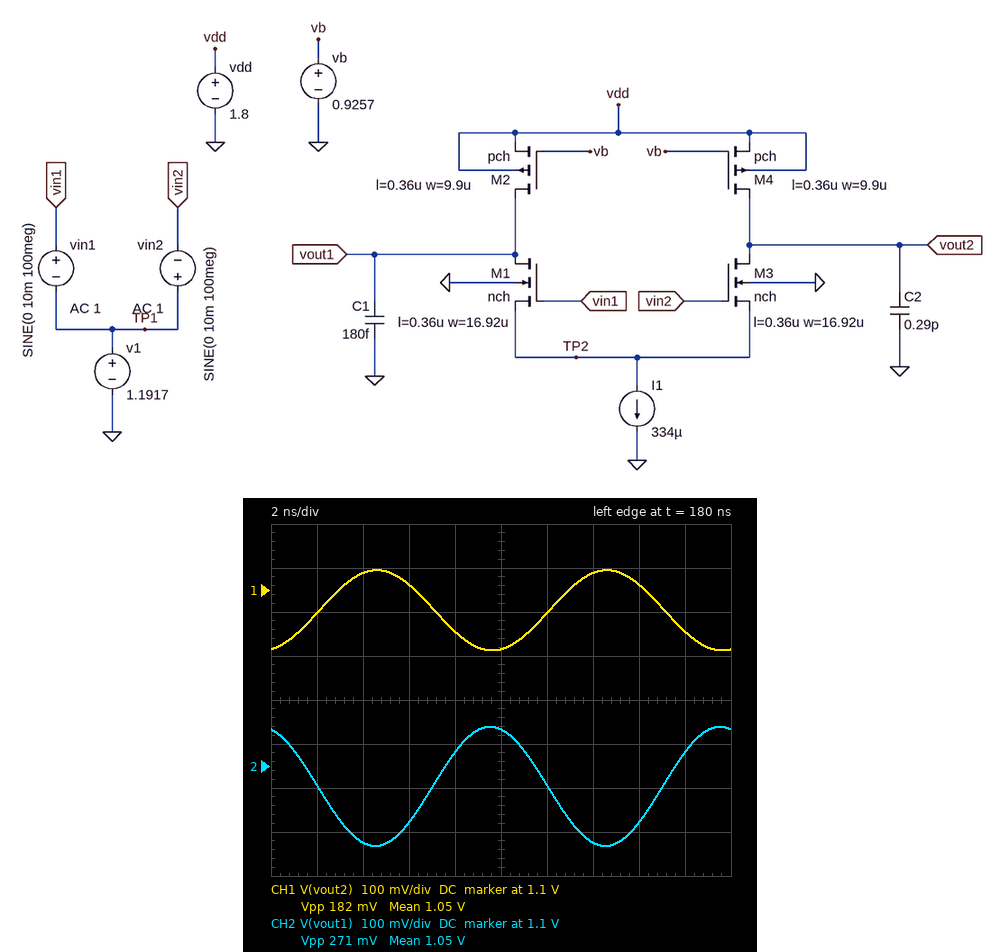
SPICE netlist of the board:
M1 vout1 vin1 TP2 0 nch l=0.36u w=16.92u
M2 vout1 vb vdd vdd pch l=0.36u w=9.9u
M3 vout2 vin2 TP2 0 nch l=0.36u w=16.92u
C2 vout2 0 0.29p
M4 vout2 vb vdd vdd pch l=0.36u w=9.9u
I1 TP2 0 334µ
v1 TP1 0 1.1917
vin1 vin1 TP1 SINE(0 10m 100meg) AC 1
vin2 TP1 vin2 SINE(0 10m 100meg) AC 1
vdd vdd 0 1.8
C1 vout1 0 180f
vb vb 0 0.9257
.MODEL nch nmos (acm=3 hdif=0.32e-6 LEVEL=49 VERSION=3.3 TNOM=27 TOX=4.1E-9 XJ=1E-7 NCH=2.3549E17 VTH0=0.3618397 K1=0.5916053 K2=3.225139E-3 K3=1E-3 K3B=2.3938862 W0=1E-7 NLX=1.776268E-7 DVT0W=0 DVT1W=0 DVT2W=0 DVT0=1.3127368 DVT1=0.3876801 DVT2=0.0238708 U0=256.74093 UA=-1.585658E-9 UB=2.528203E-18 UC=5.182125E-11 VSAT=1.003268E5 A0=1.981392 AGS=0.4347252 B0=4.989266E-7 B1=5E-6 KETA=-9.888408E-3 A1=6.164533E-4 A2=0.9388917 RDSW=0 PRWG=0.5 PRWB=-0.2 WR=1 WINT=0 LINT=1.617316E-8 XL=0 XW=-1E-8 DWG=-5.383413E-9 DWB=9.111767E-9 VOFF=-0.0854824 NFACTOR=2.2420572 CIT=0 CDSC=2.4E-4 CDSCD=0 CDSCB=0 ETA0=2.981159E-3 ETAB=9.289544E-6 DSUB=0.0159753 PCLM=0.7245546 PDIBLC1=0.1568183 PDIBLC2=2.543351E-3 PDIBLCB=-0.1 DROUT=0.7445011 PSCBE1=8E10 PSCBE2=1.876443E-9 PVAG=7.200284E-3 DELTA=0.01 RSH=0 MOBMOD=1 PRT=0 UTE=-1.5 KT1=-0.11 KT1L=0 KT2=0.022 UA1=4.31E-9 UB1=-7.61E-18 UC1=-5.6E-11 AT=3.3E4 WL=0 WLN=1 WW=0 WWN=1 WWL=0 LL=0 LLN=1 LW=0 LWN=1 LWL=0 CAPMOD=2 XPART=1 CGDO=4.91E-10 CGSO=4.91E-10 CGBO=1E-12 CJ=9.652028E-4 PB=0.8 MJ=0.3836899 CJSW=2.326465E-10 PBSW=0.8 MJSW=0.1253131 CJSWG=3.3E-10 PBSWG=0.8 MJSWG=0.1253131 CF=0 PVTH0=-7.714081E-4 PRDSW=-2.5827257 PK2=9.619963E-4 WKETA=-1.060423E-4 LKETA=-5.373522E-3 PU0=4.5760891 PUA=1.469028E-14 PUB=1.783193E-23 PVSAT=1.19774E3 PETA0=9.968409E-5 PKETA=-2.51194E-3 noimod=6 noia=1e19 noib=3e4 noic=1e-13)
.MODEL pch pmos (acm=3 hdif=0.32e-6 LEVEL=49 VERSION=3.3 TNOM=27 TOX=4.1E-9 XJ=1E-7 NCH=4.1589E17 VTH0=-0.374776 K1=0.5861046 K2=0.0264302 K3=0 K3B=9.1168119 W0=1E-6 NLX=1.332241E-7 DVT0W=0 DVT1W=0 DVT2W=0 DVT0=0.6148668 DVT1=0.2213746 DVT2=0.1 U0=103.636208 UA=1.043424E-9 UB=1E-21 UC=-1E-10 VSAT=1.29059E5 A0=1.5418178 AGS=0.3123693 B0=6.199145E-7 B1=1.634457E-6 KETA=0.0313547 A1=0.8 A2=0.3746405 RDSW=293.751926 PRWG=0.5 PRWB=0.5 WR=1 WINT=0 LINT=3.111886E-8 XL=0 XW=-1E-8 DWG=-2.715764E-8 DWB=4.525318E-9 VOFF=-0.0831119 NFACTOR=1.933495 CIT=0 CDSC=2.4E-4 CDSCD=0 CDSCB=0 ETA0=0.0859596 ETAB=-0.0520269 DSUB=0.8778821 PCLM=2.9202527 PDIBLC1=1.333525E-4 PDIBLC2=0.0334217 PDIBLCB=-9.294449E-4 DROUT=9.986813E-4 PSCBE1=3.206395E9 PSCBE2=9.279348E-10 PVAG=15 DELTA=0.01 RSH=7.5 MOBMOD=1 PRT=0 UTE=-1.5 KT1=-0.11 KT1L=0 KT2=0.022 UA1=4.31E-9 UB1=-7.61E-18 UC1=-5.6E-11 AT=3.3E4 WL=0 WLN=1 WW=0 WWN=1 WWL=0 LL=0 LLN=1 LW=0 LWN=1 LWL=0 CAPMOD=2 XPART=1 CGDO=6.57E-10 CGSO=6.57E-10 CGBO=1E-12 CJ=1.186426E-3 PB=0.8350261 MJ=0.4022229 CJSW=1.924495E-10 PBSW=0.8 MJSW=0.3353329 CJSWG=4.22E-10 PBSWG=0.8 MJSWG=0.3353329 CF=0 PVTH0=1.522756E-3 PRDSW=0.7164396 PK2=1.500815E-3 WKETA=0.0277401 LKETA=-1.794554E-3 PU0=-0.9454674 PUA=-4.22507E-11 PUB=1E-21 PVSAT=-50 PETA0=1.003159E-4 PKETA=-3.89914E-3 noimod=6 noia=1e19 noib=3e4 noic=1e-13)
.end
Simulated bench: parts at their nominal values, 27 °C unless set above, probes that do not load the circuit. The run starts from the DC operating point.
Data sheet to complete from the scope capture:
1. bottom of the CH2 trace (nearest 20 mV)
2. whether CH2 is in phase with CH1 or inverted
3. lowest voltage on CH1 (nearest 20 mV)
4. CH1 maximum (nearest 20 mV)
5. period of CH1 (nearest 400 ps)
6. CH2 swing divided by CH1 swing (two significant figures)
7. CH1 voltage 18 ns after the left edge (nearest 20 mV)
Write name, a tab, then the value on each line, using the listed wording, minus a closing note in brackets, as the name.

bottom of the CH2 trace	920 mV
whether CH2 is in phase with CH1 or inverted	inverted
lowest voltage on CH1	960 mV
CH1 maximum	1.14 V
period of CH1	10.0 ns
CH2 swing divided by CH1 swing	1.5
CH1 voltage 18 ns after the left edge	1.00 V
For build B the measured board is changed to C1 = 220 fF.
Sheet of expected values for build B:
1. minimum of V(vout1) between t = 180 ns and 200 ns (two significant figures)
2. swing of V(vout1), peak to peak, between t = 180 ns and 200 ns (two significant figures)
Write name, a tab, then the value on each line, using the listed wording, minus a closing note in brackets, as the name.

minimum of V(vout1) between t = 180 ns and 200 ns	940 mV
swing of V(vout1), peak to peak, between t = 180 ns and 200 ns	230 mV
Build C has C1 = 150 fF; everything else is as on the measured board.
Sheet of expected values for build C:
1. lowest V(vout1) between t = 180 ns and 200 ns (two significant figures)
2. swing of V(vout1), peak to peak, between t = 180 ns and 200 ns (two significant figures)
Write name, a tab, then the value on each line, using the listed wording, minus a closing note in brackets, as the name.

lowest V(vout1) between t = 180 ns and 200 ns	900 mV
swing of V(vout1), peak to peak, between t = 180 ns and 200 ns	310 mV
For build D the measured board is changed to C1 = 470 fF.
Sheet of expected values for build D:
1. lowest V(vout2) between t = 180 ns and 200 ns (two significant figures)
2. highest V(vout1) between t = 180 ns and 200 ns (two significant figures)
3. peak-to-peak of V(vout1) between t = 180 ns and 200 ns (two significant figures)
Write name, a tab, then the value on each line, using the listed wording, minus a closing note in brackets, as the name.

lowest V(vout2) between t = 180 ns and 200 ns	960 mV
highest V(vout1) between t = 180 ns and 200 ns	1.1 V
peak-to-peak of V(vout1) between t = 180 ns and 200 ns	120 mV
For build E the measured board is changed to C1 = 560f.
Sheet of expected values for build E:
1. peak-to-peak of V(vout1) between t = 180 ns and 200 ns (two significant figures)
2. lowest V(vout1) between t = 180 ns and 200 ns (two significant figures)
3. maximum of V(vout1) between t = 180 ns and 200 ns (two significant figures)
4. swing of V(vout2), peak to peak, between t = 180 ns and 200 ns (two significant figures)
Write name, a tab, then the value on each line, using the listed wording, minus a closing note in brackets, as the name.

peak-to-peak of V(vout1) between t = 180 ns and 200 ns	100 mV
lowest V(vout1) between t = 180 ns and 200 ns	1.0 V
maximum of V(vout1) between t = 180 ns and 200 ns	1.1 V
swing of V(vout2), peak to peak, between t = 180 ns and 200 ns	190 mV
